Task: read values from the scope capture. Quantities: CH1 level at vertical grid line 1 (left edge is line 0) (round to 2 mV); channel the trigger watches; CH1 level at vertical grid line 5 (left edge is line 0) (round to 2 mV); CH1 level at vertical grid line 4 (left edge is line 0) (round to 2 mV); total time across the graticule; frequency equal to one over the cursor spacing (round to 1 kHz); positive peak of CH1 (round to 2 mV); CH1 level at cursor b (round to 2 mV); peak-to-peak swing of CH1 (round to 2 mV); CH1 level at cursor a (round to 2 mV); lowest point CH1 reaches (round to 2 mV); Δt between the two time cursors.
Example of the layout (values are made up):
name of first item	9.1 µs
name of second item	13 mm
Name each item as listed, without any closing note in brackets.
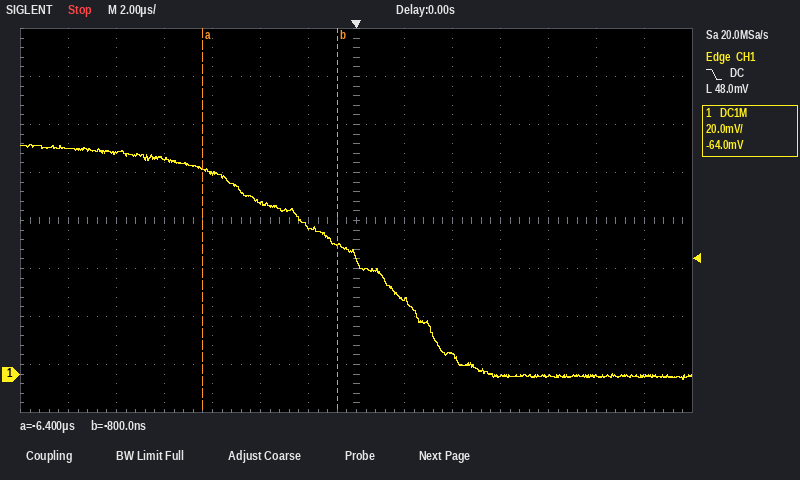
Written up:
CH1 level at vertical grid line 1 (left edge is line 0)	94 mV
channel the trigger watches	CH1
CH1 level at vertical grid line 5 (left edge is line 0)	72 mV
CH1 level at vertical grid line 4 (left edge is line 0)	84 mV
total time across the graticule	28 µs
frequency equal to one over the cursor spacing	179 kHz
positive peak of CH1	96 mV
CH1 level at cursor b	54 mV
peak-to-peak swing of CH1	98 mV
CH1 level at cursor a	86 mV
lowest point CH1 reaches	-2 mV
Δt between the two time cursors	5.6 µs
